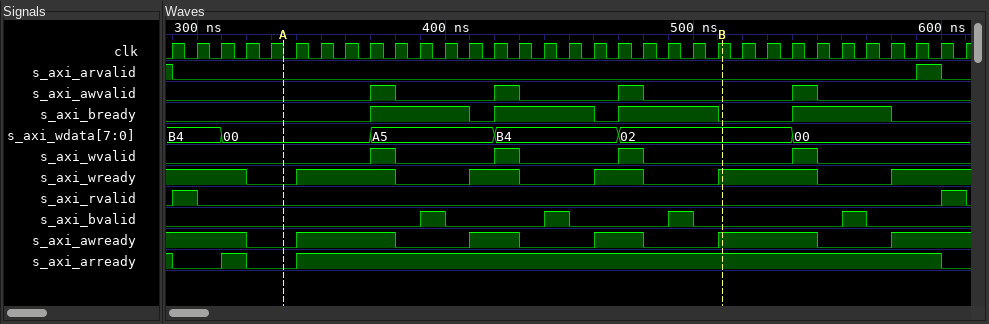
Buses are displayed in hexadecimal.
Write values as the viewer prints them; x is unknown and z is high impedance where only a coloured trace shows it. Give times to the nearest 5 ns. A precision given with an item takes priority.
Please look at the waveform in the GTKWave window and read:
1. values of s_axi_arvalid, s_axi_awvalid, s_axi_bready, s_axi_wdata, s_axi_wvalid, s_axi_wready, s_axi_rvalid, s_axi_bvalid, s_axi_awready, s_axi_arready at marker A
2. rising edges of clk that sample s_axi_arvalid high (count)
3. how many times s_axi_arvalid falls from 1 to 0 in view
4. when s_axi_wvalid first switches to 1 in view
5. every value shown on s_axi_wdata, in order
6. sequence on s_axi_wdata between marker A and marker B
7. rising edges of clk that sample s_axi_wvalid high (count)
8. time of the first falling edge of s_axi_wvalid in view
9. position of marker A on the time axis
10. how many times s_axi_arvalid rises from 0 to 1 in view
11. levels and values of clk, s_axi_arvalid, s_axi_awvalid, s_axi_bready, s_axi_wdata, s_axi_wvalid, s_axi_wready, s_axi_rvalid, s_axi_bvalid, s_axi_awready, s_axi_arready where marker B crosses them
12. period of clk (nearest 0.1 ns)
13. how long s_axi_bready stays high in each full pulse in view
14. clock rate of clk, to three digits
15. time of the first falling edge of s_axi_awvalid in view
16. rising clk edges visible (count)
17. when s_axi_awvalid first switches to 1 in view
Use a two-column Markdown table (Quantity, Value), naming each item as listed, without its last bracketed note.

| Quantity | Value |
|---|---|
| values of s_axi_arvalid, s_axi_awvalid, s_axi_bready, s_axi_wdata, s_axi_wvalid, s_axi_wready, s_axi_rvalid, s_axi_bvalid, s_axi_awready, s_axi_arready at marker A | s_axi_arvalid=0, s_axi_awvalid=0, s_axi_bready=0, s_axi_wdata=00, s_axi_wvalid=0, s_axi_wready=0, s_axi_rvalid=0, s_axi_bvalid=0, s_axi_awready=0, s_axi_arready=0 |
| rising edges of clk that sample s_axi_arvalid high | 2 |
| how many times s_axi_arvalid falls from 1 to 0 in view | 2 |
| when s_axi_wvalid first switches to 1 in view | 370 ns |
| every value shown on s_axi_wdata, in order | B4, 00, A5, B4, 02, 00 |
| sequence on s_axi_wdata between marker A and marker B | 00, A5, B4, 02 |
| rising edges of clk that sample s_axi_wvalid high | 4 |
| time of the first falling edge of s_axi_wvalid in view | 380 ns |
| position of marker A on the time axis | 335 ns |
| how many times s_axi_arvalid rises from 0 to 1 in view | 1 |
| levels and values of clk, s_axi_arvalid, s_axi_awvalid, s_axi_bready, s_axi_wdata, s_axi_wvalid, s_axi_wready, s_axi_rvalid, s_axi_bvalid, s_axi_awready, s_axi_arready where marker B crosses them | clk=1, s_axi_arvalid=0, s_axi_awvalid=0, s_axi_bready=0, s_axi_wdata=02, s_axi_wvalid=0, s_axi_wready=1, s_axi_rvalid=0, s_axi_bvalid=0, s_axi_awready=1, s_axi_arready=1 |
| period of clk | 10 ns |
| how long s_axi_bready stays high in each full pulse in view | 40 ns, 40 ns, 40 ns, 40 ns |
| clock rate of clk, to three digits | 100 MHz |
| time of the first falling edge of s_axi_awvalid in view | 380 ns |
| rising clk edges visible | 33 |
| when s_axi_awvalid first switches to 1 in view | 370 ns |
